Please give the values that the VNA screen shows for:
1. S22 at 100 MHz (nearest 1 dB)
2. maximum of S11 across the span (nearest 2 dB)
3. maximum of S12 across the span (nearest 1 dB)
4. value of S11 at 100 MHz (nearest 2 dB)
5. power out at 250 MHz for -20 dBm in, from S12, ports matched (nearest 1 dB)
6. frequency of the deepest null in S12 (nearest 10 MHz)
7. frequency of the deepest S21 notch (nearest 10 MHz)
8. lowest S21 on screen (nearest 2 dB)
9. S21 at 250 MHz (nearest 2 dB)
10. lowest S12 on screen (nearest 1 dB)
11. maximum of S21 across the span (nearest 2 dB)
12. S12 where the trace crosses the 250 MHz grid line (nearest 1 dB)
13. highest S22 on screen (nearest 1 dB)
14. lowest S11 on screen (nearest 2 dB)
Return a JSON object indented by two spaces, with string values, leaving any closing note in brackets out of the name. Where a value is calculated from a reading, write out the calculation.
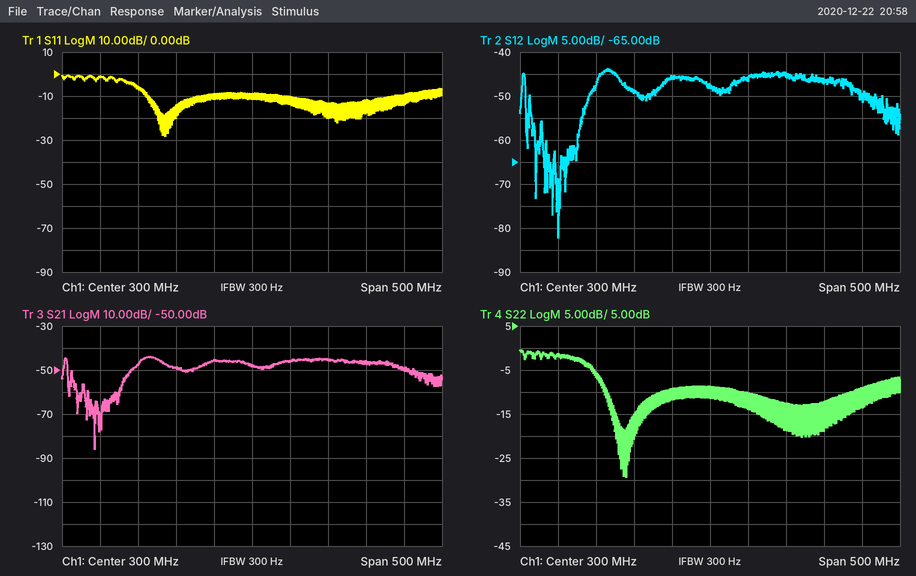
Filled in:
{
  "S22 at 100 MHz": "-2 dB",
  "maximum of S11 across the span": "0 dB",
  "maximum of S12 across the span": "-44 dB",
  "value of S11 at 100 MHz": "-2 dB",
  "power out at 250 MHz for -20 dBm in, from S12, ports matched": "-20 dBm + (-46 dB) = -66 dBm",
  "frequency of the deepest null in S12": "100 MHz",
  "frequency of the deepest S21 notch": "90 MHz",
  "lowest S21 on screen": "-86 dB",
  "S21 at 250 MHz": "-46 dB",
  "lowest S12 on screen": "-82 dB",
  "maximum of S21 across the span": "-44 dB",
  "S12 where the trace crosses the 250 MHz grid line": "-46 dB",
  "highest S22 on screen": "0 dB",
  "lowest S11 on screen": "-28 dB"
}
